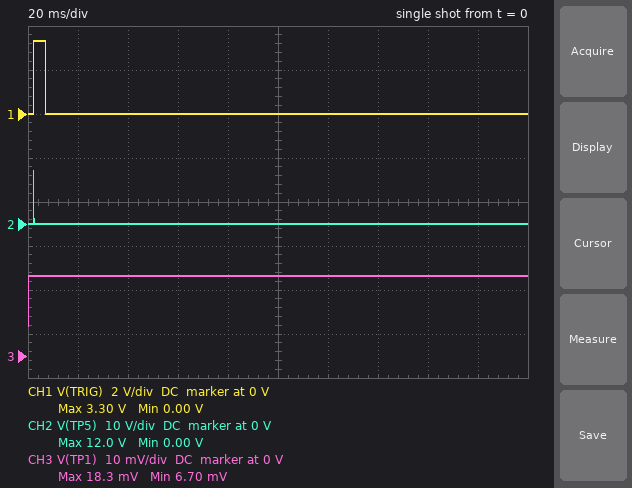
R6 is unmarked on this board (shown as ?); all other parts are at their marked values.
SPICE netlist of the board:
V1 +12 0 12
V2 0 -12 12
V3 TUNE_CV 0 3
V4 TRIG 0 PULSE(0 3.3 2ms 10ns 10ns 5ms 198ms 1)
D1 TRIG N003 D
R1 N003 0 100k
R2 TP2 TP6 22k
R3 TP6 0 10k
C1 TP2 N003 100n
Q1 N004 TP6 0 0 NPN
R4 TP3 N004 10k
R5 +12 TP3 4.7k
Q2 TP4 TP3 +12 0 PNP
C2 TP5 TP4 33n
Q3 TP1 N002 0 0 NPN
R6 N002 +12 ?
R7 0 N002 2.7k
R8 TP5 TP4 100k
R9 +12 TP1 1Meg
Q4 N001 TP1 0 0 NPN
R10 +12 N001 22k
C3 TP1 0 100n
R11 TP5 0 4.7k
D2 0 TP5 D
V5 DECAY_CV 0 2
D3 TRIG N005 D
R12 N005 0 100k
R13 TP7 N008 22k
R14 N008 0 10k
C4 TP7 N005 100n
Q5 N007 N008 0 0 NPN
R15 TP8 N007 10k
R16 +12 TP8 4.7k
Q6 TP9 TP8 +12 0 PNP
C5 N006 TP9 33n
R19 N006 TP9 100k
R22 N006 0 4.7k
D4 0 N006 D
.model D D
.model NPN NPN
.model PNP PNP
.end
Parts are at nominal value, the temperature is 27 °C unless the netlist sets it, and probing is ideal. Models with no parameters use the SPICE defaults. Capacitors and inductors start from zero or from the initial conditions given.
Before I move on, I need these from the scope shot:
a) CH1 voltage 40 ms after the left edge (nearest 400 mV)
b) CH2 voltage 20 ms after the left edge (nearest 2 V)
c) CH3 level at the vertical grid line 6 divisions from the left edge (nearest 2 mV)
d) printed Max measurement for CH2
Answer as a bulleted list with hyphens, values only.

- 0 V
- 0 V
- 18 mV
- 12.0 V
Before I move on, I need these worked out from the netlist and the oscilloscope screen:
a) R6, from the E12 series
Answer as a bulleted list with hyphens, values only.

- 15 kΩ
